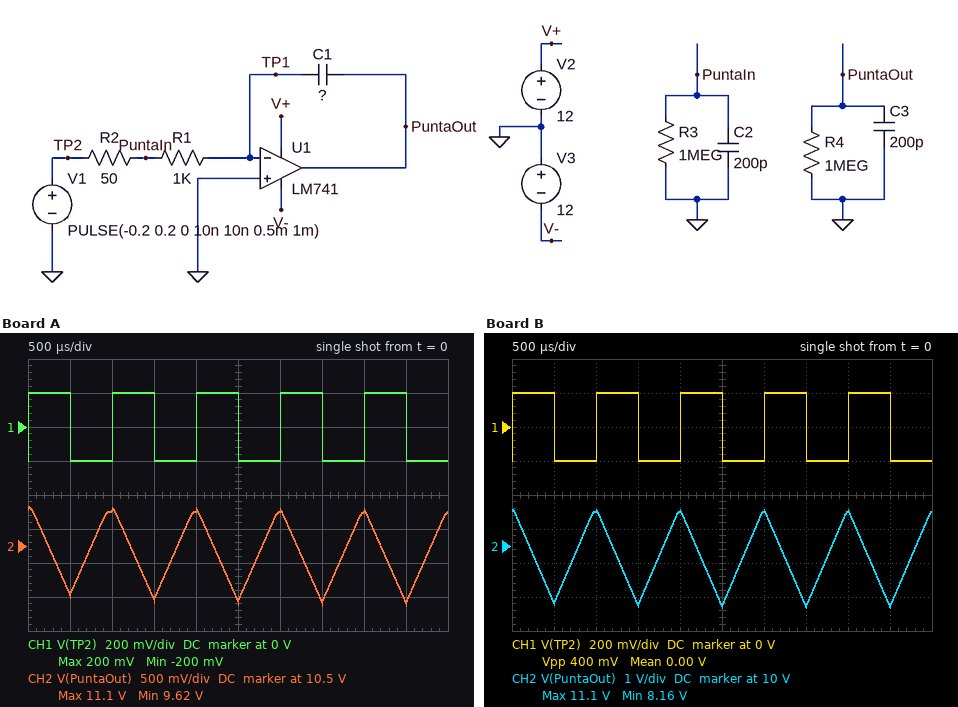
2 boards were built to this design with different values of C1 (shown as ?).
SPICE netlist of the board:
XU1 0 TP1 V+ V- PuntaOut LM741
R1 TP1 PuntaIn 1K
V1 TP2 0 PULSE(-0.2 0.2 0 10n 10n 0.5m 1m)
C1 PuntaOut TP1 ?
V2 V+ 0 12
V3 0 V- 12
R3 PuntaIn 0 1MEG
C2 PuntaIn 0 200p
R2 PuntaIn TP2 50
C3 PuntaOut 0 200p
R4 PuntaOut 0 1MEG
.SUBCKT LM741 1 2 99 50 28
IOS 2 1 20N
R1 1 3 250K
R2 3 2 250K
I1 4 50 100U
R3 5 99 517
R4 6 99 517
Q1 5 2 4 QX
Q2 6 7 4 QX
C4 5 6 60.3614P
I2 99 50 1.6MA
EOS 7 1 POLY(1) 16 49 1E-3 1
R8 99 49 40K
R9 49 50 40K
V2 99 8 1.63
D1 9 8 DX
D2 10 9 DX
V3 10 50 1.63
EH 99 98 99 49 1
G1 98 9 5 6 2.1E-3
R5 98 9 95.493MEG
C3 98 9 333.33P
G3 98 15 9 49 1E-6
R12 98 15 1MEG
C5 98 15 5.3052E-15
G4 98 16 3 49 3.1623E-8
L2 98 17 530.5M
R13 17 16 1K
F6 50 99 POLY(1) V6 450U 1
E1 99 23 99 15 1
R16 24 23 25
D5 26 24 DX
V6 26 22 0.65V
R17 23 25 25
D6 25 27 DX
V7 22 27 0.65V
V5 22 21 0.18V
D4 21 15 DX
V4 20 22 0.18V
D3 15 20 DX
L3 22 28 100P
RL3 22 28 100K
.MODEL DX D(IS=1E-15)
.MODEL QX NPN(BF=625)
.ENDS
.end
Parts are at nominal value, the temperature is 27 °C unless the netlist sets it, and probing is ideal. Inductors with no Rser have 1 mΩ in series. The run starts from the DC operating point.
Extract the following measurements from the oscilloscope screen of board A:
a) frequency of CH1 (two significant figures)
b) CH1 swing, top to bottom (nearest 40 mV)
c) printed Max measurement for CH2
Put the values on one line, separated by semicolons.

1.0 kHz; 400 mV; 11.1 V
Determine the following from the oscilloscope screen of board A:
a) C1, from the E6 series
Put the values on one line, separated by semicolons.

68 nF
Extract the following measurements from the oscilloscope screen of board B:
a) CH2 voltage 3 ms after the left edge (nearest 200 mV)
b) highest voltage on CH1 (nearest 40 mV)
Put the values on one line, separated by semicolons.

11.0 V; 200 mV
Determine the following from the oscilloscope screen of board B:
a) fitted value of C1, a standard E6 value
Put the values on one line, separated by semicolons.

33 nF
